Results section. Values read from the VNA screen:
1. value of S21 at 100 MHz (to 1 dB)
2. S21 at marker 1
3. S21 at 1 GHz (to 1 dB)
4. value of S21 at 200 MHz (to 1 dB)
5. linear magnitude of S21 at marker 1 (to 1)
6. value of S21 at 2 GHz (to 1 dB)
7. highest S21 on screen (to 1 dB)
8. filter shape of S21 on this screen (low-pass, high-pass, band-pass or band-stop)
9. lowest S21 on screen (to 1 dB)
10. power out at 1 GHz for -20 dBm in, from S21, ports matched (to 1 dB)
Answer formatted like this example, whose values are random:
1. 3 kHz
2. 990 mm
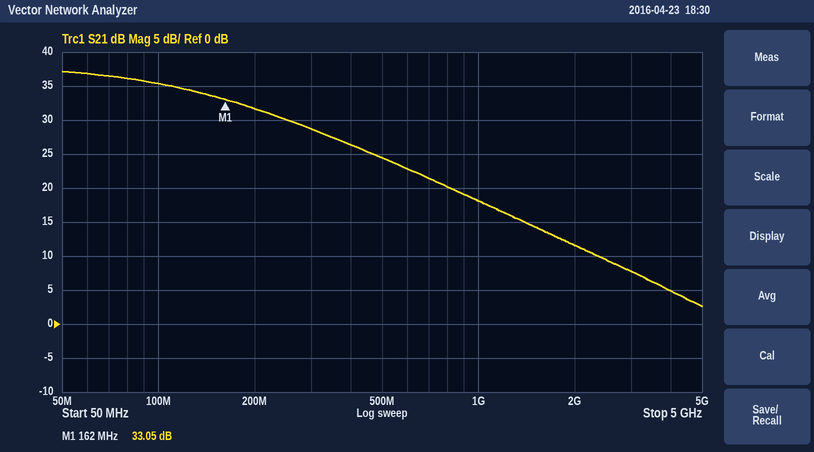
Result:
1. 35 dB
2. 33.05 dB
3. 18 dB
4. 32 dB
5. 45
6. 12 dB
7. 37 dB
8. low-pass
9. 3 dB
10. -2 dBm
